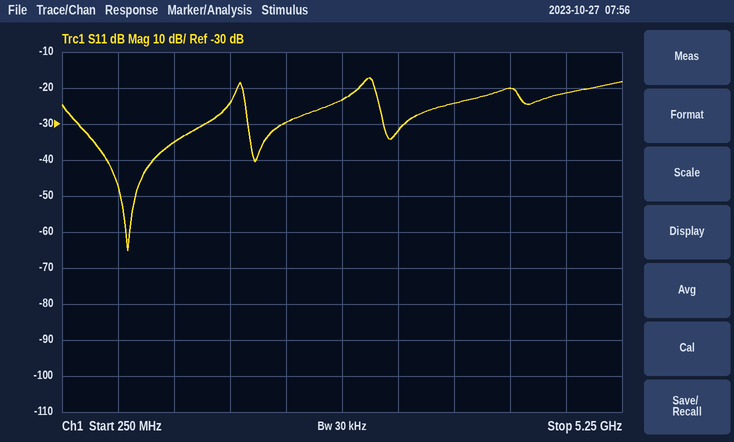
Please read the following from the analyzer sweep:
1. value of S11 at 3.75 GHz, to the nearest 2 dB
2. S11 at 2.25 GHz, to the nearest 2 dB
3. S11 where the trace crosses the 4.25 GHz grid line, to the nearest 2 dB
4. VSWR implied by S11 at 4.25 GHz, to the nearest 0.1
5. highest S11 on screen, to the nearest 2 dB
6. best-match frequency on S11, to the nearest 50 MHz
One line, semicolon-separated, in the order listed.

-24 dB; -30 dB; -20 dB; 1.2; -18 dB; 850 MHz
